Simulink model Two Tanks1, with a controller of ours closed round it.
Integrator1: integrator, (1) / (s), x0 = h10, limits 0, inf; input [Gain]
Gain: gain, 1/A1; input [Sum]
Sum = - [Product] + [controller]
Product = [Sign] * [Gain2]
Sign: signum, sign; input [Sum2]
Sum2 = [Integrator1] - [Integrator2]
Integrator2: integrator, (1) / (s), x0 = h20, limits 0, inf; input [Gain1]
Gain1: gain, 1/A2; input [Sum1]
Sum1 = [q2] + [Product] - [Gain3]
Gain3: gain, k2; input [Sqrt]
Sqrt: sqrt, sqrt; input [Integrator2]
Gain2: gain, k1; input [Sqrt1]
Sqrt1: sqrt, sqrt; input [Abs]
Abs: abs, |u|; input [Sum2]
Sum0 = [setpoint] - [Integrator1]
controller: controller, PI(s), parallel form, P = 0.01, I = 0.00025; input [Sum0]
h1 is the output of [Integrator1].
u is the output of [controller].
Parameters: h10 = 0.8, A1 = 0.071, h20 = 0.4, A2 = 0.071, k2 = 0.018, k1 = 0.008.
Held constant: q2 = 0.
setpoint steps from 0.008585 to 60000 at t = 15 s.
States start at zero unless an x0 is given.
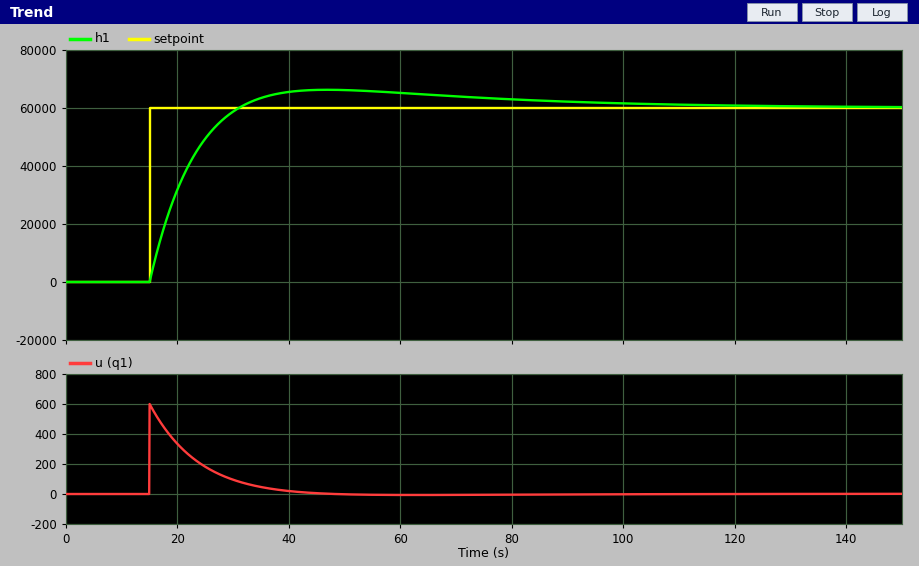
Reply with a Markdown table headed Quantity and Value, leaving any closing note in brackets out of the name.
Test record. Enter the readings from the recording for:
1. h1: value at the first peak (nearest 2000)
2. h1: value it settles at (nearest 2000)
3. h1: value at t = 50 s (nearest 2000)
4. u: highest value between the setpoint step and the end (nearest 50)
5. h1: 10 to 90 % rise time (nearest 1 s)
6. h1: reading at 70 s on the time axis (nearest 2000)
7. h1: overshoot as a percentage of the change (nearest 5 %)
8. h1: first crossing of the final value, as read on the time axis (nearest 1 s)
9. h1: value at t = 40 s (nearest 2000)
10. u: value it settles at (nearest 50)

| Quantity | Value |
|---|---|
| h1: value at the first peak | 66000 |
| h1: value it settles at | 60000 |
| h1: value at t = 50 s | 66000 |
| u: highest value between the setpoint step and the end | 600 |
| h1: 10 to 90 % rise time | 11 s |
| h1: reading at 70 s on the time axis | 64000 |
| h1: overshoot as a percentage of the change | 10 % |
| h1: first crossing of the final value, as read on the time axis | 31 s |
| h1: value at t = 40 s | 66000 |
| u: value it settles at | 0 |
